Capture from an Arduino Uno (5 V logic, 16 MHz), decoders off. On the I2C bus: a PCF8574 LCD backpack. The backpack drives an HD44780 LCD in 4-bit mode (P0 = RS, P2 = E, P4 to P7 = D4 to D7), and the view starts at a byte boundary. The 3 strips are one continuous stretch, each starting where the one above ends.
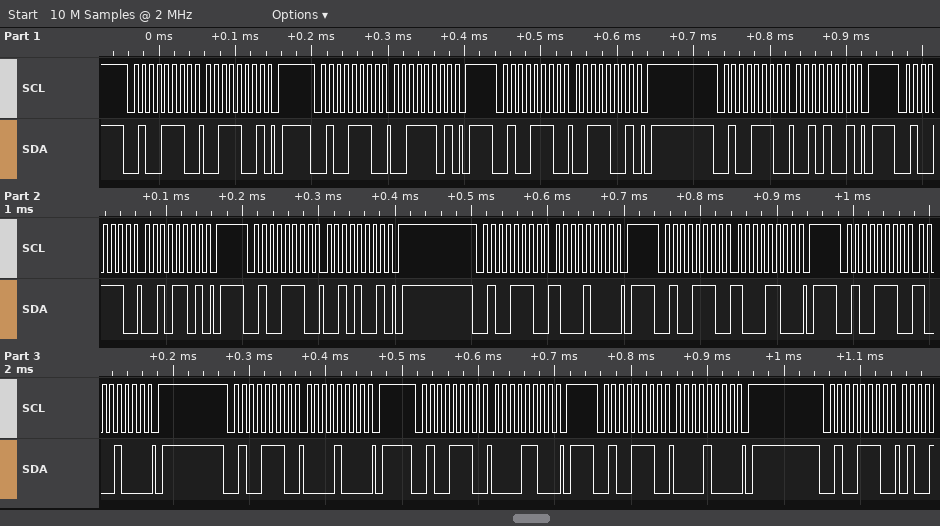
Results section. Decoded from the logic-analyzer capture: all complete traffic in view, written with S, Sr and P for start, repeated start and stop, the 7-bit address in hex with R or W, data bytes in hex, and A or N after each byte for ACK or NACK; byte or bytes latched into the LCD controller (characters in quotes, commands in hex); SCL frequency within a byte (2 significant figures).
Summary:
S 27W A 39 A P S 27W A 3D A P S 27W A 39 A P S 27W A 29 A P S 27W A 2D A P S 27W A 29 A P S 27W A 88 A P S 27W A 8C A P S 27W A 88 A P S 27W A 08 A P S 27W A 0C A P S 27W A 08 A P S 27W A
'2' 0x80
100 kHz
